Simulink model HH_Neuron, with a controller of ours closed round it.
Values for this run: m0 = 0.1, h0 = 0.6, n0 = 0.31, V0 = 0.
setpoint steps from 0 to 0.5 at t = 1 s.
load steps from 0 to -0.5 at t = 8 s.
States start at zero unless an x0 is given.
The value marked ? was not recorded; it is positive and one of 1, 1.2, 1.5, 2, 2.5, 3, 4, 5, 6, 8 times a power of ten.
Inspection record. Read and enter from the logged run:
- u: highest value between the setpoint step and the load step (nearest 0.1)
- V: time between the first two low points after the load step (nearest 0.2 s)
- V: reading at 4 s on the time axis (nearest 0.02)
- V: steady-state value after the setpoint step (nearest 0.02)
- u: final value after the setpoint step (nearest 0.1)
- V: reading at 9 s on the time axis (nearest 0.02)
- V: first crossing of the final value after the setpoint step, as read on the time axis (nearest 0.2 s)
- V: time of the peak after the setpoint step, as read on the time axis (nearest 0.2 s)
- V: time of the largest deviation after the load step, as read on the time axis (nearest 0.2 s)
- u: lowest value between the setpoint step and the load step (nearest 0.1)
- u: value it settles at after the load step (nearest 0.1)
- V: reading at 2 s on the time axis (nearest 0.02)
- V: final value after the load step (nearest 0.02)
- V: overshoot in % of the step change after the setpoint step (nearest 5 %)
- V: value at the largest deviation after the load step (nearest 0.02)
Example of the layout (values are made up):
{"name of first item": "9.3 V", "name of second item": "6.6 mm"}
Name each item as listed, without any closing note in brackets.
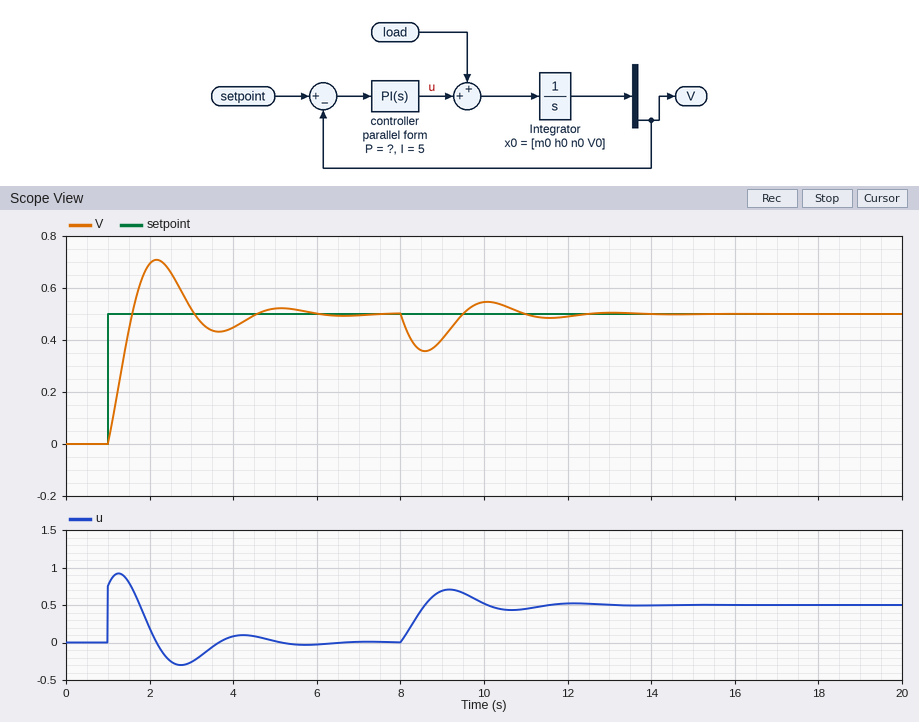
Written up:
{"u: highest value between the setpoint step and the load step": "0.9", "V: time between the first two low points after the load step": "3.0 s", "V: reading at 4 s on the time axis": "0.44", "V: steady-state value after the setpoint step": "0.50", "u: final value after the setpoint step": "0.0", "V: reading at 9 s on the time axis": "0.40", "V: first crossing of the final value after the setpoint step, as read on the time axis": "1.6 s", "V: time of the peak after the setpoint step, as read on the time axis": "2.2 s", "V: time of the largest deviation after the load step, as read on the time axis": "8.6 s", "u: lowest value between the setpoint step and the load step": "-0.3", "u: value it settles at after the load step": "0.5", "V: reading at 2 s on the time axis": "0.70", "V: final value after the load step": "0.50", "V: overshoot in % of the step change after the setpoint step": "40 %", "V: value at the largest deviation after the load step": "0.36"}
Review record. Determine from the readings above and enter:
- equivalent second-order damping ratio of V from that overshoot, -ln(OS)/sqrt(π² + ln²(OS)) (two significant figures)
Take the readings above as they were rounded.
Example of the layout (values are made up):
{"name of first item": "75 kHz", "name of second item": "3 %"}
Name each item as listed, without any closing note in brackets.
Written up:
{"equivalent second-order damping ratio of V from that overshoot, -ln(OS)/sqrt(π² + ln²(OS))": "0.28"}
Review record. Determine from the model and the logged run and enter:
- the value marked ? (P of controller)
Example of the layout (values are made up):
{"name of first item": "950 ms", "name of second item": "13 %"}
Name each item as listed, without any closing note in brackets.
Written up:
{"the value marked ?": "1.5"}
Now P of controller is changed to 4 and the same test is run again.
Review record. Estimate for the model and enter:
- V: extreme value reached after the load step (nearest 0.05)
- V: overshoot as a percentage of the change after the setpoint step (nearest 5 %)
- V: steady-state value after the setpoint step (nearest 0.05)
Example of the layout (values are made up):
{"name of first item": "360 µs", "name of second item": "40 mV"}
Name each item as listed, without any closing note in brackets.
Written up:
{"V: extreme value reached after the load step": "0.40", "V: overshoot as a percentage of the change after the setpoint step": "15 %", "V: steady-state value after the setpoint step": "0.50"}
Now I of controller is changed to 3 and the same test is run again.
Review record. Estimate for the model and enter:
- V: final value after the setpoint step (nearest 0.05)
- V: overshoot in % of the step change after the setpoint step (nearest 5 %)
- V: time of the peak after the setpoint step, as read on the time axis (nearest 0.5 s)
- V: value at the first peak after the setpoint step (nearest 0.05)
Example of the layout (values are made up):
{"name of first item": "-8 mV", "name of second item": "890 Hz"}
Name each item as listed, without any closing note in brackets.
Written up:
{"V: final value after the setpoint step": "0.50", "V: overshoot in % of the step change after the setpoint step": "35 %", "V: time of the peak after the setpoint step, as read on the time axis": "2.5 s", "V: value at the first peak after the setpoint step": "0.65"}
